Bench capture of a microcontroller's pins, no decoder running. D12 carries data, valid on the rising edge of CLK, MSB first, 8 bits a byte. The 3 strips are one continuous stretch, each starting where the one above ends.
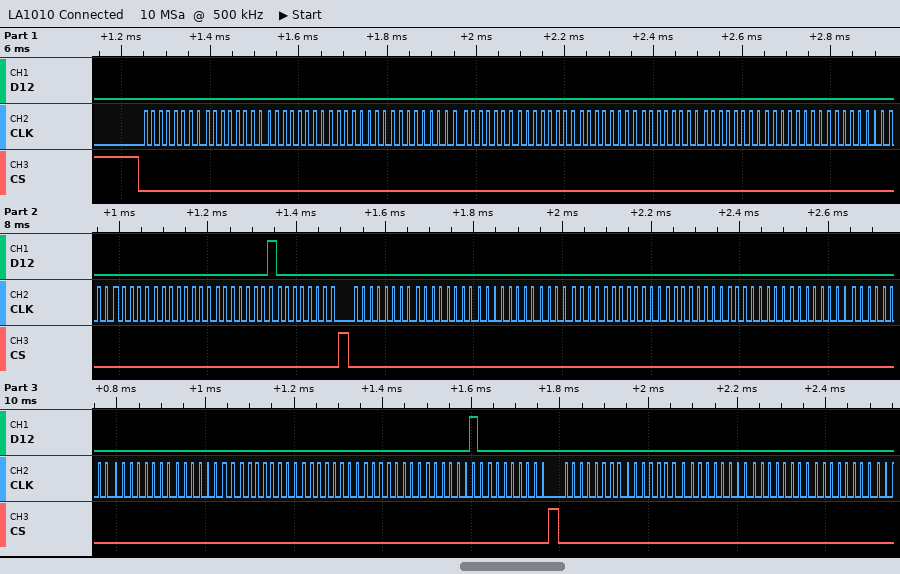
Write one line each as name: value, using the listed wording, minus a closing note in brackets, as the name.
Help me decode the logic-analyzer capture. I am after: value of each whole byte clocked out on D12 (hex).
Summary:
value of each whole byte clocked out on D12: 00 00 00 00 00 00 00 00 00 00 00 00 00 00 01 00 00 00 00 00 00 00 00 00 00 00 00 00 00 00 02 00 00 00 00 00 00
